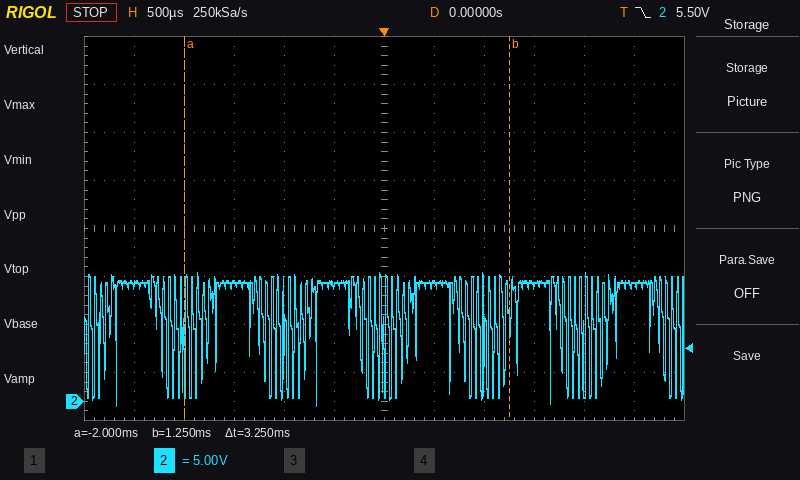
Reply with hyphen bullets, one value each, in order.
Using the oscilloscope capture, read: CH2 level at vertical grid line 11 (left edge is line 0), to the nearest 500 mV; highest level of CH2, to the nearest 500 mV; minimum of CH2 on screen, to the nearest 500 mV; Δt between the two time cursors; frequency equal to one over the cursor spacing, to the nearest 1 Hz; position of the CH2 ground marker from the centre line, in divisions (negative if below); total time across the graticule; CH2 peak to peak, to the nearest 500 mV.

- 12.0 V
- 13.5 V
- -500 mV
- 3.25 ms
- 308 Hz
- -3.6 div
- 6 ms
- 14.0 V
